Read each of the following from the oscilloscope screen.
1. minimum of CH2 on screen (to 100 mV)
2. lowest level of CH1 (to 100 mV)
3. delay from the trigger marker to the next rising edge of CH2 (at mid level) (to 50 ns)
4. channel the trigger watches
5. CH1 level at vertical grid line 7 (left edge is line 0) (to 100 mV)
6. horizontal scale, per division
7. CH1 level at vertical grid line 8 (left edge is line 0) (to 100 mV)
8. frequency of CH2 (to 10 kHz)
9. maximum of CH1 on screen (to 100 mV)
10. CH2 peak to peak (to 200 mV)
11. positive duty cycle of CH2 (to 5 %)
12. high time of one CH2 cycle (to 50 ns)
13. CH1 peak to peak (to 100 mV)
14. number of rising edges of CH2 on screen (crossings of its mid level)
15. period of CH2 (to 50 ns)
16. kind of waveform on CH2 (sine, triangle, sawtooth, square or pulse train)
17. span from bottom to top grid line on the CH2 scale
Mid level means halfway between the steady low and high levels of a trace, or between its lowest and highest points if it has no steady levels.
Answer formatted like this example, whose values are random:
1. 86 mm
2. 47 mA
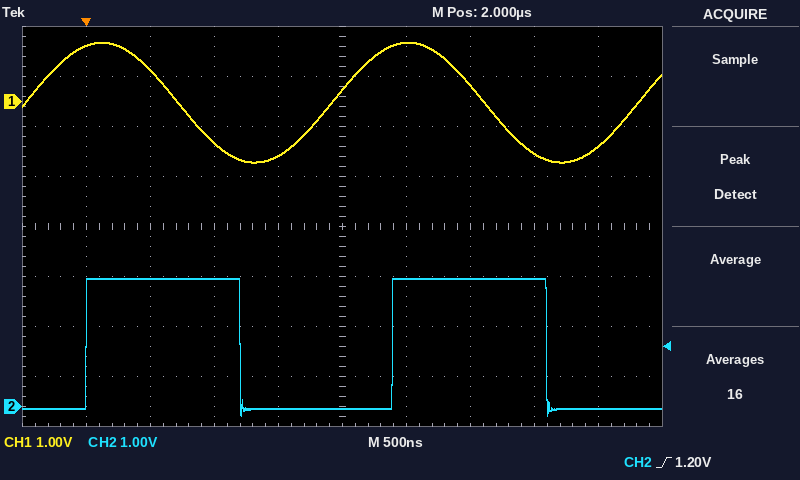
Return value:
1. -200 mV
2. -1.2 V
3. 2.40 µs
4. CH2
5. 300 mV
6. 500 ns
7. -1.0 V
8. 420 kHz
9. 1.2 V
10. 2.8 V
11. 50 %
12. 1.20 µs
13. 2.4 V
14. 2
15. 2.40 µs
16. square
17. 8 V
